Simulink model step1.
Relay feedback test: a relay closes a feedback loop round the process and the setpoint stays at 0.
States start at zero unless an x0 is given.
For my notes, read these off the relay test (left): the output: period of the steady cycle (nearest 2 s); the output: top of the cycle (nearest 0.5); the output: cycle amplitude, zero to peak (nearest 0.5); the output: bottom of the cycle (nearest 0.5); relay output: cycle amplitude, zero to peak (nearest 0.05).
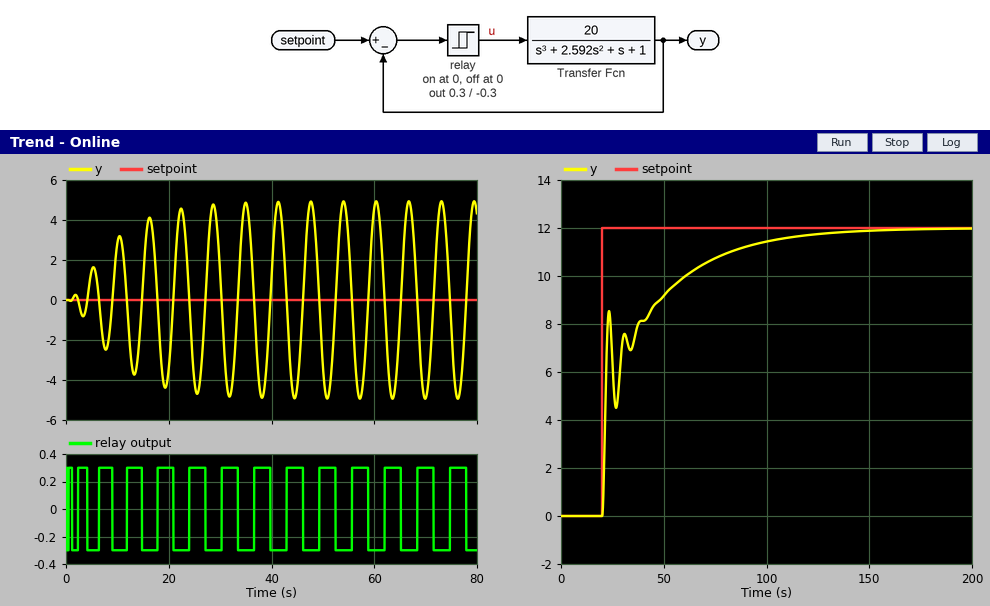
6 s
5.0
5.0
-5.0
0.30
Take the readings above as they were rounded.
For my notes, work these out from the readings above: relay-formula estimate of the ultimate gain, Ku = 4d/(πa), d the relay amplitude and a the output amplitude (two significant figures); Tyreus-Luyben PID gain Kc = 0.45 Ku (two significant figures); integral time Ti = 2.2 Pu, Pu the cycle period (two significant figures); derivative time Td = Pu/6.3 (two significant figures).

0.076
0.034
13 s
0.95 s
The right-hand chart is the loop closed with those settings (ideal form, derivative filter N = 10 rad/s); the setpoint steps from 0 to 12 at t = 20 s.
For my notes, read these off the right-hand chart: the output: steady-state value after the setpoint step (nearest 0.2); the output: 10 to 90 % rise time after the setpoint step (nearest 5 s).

12.0
55 s
